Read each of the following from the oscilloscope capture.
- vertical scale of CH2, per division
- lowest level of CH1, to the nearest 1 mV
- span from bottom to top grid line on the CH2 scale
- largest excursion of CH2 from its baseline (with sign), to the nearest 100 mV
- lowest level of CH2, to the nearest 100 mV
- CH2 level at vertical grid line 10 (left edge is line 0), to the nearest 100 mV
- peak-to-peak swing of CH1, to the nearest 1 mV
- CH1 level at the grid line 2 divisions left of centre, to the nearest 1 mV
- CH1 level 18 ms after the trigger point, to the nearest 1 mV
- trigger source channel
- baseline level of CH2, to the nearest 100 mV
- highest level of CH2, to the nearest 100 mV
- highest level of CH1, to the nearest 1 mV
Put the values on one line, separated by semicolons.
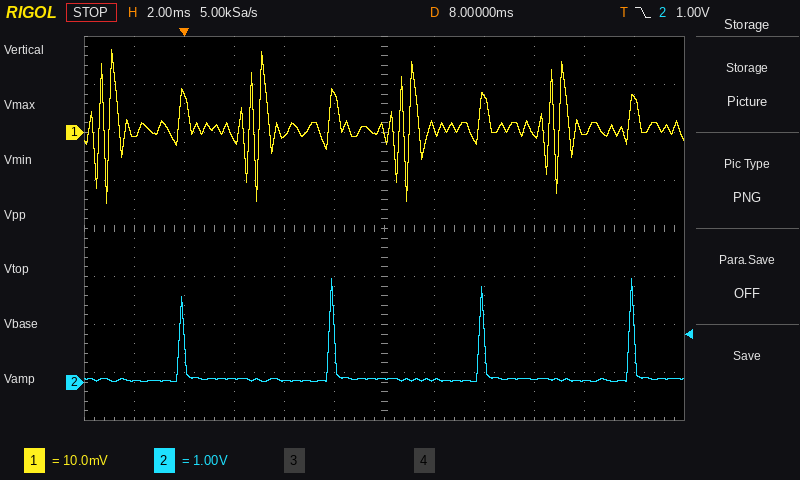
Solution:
1 V; -15 mV; 8 V; +2.1 V; 0.0 V; 0.0 V; 32 mV; -1 mV; 7 mV; CH2; 100 mV; 2.2 V; 17 mV
